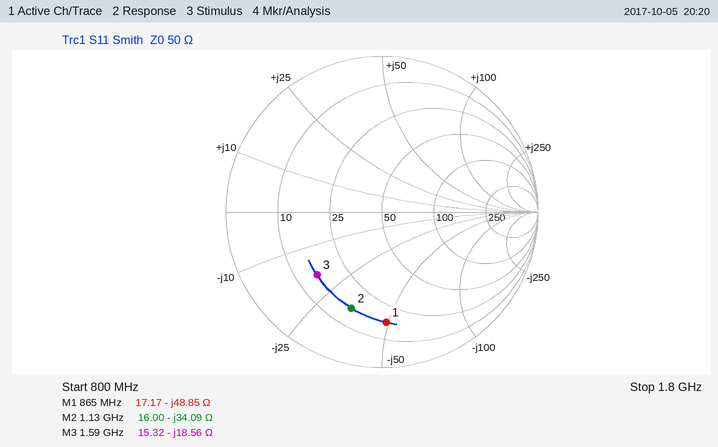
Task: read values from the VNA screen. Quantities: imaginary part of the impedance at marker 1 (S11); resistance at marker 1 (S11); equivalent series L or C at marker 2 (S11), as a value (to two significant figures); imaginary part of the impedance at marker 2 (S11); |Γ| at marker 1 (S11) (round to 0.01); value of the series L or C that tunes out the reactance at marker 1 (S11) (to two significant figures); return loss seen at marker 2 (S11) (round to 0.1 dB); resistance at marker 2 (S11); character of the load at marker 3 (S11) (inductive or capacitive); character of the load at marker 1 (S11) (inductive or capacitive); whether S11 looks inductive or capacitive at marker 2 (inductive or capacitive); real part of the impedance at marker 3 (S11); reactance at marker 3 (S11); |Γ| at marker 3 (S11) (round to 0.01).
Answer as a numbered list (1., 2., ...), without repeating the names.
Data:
1. -48.85 Ω
2. 17.17 Ω
3. 4.1 pF
4. -34.09 Ω
5. 0.71
6. 9.0 nH
7. 3.8 dB
8. 16.00 Ω
9. capacitive
10. capacitive
11. capacitive
12. 15.32 Ω
13. -18.56 Ω
14. 0.58
